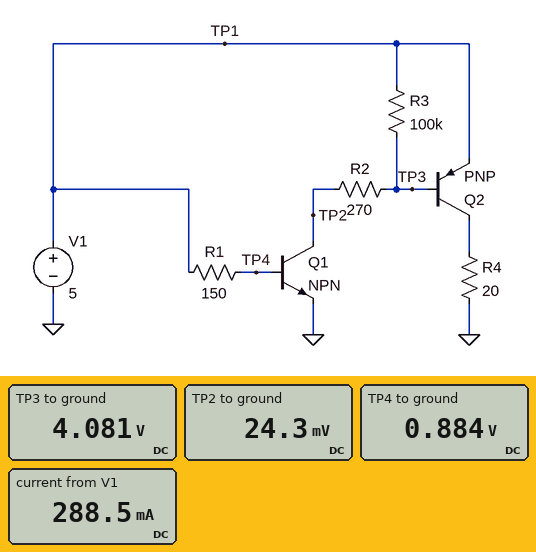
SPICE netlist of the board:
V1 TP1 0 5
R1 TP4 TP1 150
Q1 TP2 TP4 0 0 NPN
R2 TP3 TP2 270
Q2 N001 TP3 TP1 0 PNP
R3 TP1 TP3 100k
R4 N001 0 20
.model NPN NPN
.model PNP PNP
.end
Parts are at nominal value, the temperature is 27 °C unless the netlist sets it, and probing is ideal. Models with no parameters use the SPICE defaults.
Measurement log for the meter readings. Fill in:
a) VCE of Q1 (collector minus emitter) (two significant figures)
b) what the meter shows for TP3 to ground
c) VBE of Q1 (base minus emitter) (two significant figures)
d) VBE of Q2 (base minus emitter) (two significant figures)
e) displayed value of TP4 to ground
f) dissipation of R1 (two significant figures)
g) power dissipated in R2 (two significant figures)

24 mV
4.081 V
880 mV
-920 mV
0.884 V
110 mW
61 mW
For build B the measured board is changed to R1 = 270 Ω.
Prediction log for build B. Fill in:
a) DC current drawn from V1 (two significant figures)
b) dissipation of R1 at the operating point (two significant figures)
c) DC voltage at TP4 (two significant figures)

280 mA
63 mW
870 mV
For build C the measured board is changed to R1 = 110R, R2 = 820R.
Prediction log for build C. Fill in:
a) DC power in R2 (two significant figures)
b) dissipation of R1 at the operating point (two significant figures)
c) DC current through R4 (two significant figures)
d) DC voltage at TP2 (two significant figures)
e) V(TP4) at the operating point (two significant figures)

20 mW
150 mW
240 mA
20 mV
890 mV
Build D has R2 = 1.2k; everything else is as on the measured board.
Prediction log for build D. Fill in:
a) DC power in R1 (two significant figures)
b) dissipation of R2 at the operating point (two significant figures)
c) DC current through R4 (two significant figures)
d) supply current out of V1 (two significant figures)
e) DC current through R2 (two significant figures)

110 mW
14 mW
240 mA
270 mA
3.4 mA
